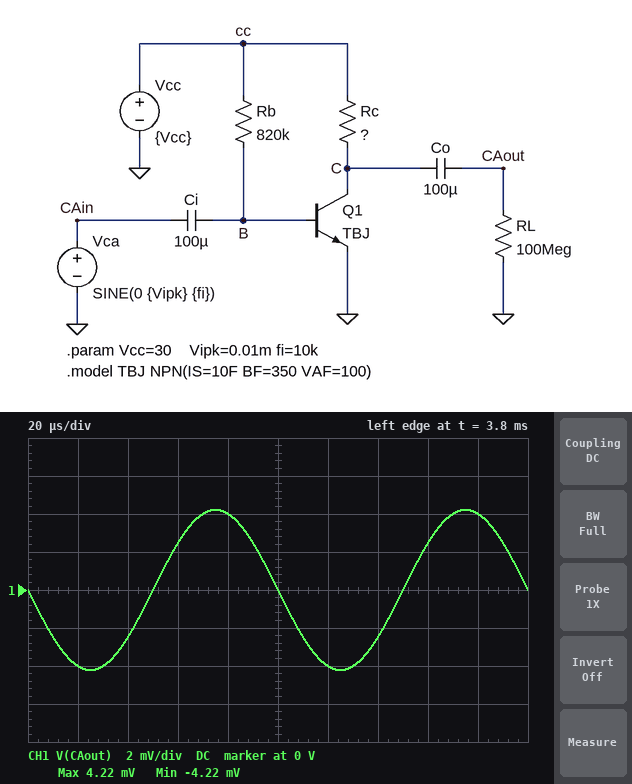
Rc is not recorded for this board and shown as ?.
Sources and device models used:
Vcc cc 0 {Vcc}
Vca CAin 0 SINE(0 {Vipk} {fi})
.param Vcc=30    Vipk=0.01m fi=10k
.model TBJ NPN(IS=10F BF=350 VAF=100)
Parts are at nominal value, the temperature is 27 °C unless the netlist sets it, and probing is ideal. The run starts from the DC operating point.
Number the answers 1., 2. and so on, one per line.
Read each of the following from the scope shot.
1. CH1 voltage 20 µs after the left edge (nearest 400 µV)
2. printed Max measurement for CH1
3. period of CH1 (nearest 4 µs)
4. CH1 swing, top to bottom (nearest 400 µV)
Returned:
1. -4.0 mV
2. 4.22 mV
3. 100 µs
4. 8.4 mV
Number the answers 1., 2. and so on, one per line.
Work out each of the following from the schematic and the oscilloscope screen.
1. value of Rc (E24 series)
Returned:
1. 820 Ω
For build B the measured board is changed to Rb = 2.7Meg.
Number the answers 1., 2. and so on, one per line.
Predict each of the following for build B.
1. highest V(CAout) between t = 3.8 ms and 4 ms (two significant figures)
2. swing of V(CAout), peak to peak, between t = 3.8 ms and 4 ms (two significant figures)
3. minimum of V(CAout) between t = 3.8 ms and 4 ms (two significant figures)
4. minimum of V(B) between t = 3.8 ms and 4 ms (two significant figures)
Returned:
1. 1.5 mV
2. 2.9 mV
3. -1.5 mV
4. 690 mV
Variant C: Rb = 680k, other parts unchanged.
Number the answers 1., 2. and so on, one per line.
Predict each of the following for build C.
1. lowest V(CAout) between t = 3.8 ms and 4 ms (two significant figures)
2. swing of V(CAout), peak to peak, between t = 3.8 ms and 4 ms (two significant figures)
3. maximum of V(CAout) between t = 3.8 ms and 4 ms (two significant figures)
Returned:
1. -4.9 mV
2. 9.8 mV
3. 4.9 mV
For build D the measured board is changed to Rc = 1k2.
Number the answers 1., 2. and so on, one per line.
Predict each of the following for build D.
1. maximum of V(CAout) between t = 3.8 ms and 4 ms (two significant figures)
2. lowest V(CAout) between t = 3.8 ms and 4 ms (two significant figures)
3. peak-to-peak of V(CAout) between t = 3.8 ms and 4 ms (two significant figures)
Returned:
1. 5.7 mV
2. -5.7 mV
3. 11 mV
